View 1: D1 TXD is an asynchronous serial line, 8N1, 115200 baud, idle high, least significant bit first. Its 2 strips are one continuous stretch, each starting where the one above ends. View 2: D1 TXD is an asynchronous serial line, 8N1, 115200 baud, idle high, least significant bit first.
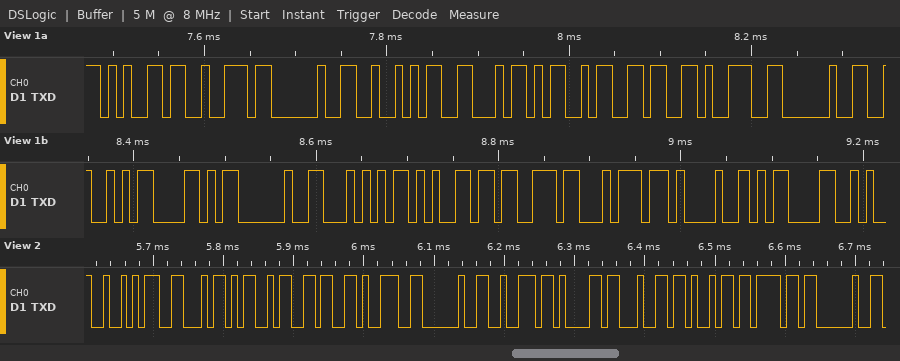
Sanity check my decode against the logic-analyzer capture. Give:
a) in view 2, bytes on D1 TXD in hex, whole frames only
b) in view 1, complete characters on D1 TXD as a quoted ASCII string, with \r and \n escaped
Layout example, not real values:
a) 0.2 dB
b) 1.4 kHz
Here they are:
a) 0x52 0x46 0x4D 0x36 0x39 0x20 0x72 0x61 0x64 0x69 0x6F 0x20
b) "er RFM69 RX Test!\r"
